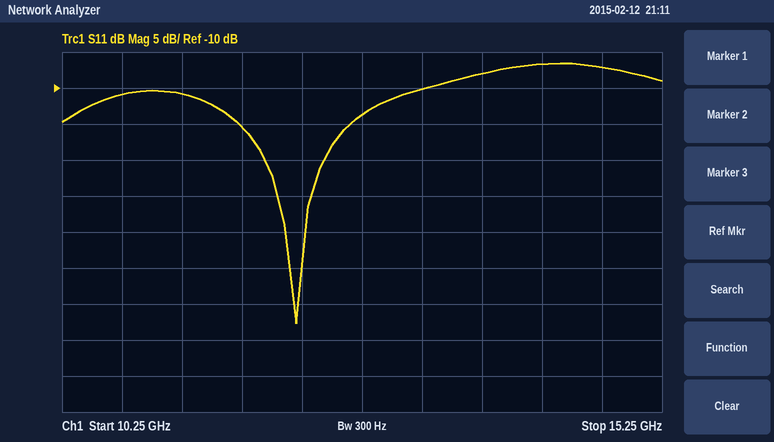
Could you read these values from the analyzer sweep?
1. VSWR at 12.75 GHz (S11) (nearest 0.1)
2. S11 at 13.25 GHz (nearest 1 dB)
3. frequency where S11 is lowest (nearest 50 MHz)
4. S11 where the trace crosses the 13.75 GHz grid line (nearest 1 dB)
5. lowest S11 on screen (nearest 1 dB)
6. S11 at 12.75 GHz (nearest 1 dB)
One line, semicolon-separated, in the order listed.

1.5; -10 dB; 12.20 GHz; -8 dB; -43 dB; -14 dB
